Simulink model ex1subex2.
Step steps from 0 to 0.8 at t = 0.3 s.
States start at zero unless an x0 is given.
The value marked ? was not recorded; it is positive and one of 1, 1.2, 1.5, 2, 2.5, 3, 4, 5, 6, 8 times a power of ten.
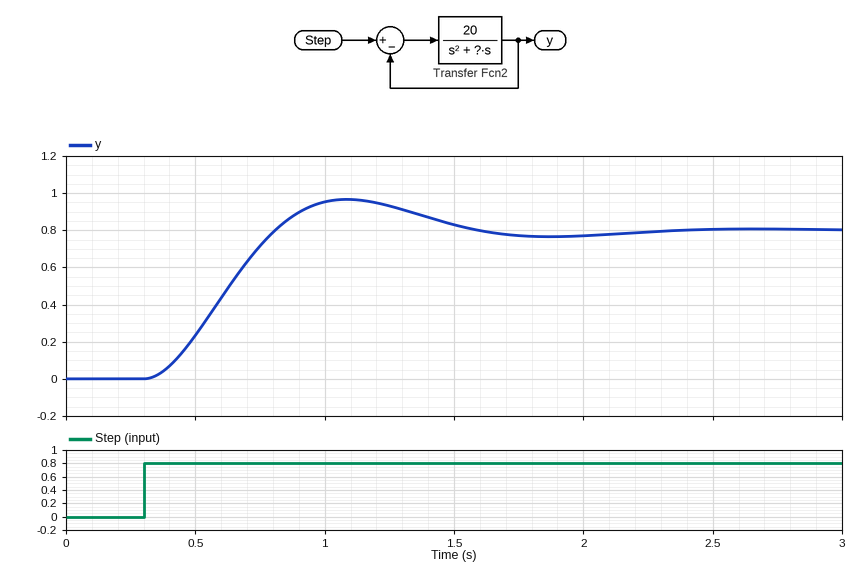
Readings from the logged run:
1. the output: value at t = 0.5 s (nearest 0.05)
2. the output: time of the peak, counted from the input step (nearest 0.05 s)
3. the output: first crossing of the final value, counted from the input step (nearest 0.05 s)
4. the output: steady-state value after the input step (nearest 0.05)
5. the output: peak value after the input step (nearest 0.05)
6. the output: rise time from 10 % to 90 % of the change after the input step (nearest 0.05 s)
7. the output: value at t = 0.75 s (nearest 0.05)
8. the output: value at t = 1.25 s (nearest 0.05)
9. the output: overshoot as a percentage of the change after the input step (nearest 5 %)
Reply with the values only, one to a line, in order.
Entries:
0.25
0.80 s
0.50 s
0.80
0.95
0.35 s
0.70
0.95
20 %
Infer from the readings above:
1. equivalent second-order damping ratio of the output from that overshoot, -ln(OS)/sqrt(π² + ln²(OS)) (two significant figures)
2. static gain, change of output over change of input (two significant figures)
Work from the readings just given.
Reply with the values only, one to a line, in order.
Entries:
0.46
1.0
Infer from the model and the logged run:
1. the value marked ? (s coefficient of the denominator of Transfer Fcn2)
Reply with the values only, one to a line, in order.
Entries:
4
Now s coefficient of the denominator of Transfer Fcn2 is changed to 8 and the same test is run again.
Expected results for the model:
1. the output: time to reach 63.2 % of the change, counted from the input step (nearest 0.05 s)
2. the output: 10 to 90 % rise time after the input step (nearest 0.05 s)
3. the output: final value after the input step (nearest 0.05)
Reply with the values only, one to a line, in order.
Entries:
0.45 s
0.65 s
0.80
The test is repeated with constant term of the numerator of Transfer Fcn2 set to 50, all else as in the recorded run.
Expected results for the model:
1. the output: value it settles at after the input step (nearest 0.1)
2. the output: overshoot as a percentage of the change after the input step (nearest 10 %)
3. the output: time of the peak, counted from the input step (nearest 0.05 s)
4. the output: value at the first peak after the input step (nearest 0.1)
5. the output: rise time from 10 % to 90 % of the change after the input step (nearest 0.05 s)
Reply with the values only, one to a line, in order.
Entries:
0.8
40 %
0.45 s
1.1
0.20 s
